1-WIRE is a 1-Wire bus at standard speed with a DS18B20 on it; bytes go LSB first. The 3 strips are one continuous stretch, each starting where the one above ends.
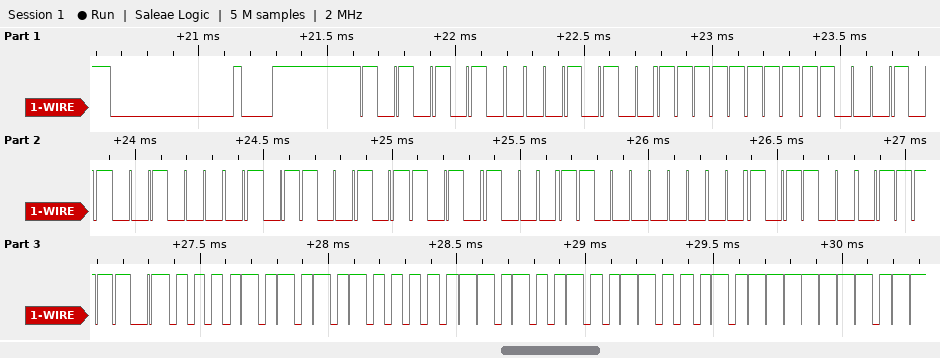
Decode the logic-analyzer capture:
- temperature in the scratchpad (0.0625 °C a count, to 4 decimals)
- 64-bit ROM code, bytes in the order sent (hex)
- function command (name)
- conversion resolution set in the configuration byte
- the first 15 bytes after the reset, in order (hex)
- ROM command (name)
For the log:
85.0000 °C
28 FF A3 84 A6 15 03 34
Read Scratchpad
12 bits
55 28 FF A3 84 A6 15 03 34 BE 50 05 4B 46 7F
Match ROM
